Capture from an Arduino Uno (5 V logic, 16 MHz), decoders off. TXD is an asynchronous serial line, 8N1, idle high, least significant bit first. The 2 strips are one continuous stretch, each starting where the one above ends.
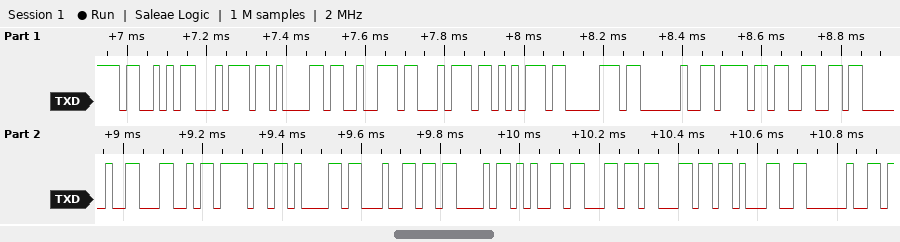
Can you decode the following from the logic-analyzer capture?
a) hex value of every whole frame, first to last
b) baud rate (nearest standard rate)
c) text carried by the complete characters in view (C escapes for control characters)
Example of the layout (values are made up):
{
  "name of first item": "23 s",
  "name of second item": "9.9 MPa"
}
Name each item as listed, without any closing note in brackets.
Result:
{
  "hex value of every whole frame, first to last": "0x53 0x74 0x61 0x72 0x74 0x75 0x70 0x20 0x6F 0x66 0x20 0x4C 0x6F 0x61 0x64 0x43 0x65 0x6C 0x6C 0x31 0x20",
  "baud rate": "57600 baud",
  "text carried by the complete characters in view": "\"Startup of LoadCell1 \""
}
